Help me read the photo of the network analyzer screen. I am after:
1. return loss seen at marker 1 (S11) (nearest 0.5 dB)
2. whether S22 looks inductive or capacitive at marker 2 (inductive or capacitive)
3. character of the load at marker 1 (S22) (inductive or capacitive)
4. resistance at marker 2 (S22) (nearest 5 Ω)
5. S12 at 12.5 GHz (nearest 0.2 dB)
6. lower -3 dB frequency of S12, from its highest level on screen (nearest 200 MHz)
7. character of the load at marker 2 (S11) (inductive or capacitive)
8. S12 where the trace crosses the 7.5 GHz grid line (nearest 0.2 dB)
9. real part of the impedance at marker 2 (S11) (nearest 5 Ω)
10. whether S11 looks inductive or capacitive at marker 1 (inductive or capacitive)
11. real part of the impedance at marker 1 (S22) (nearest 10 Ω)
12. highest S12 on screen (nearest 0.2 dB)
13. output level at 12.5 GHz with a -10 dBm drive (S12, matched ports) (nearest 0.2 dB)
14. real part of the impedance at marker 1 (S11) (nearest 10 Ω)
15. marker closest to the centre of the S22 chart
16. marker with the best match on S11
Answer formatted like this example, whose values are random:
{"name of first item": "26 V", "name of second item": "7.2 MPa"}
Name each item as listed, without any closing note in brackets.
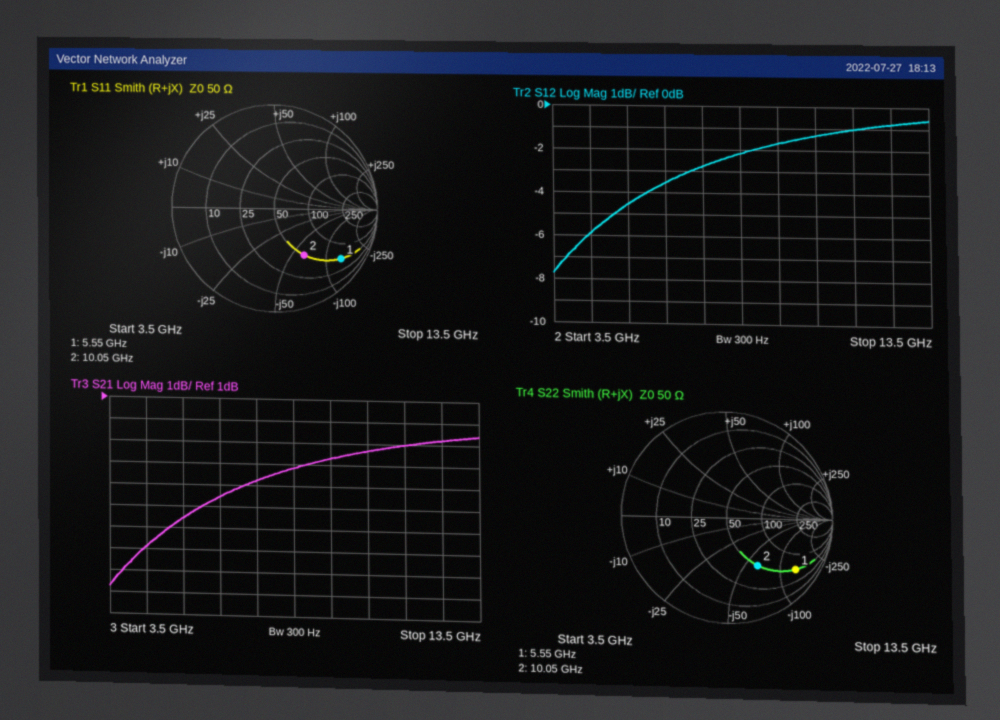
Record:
{"return loss seen at marker 1 (S11)": "2.0 dB", "whether S22 looks inductive or capacitive at marker 2": "capacitive", "character of the load at marker 1 (S22)": "capacitive", "resistance at marker 2 (S22)": "50 Ω", "S12 at 12.5 GHz": "-0.8 dB", "lower -3 dB frequency of S12, from its highest level on screen": "6.4 GHz", "character of the load at marker 2 (S11)": "capacitive", "S12 where the trace crosses the 7.5 GHz grid line": "-2.8 dB", "real part of the impedance at marker 2 (S11)": "50 Ω", "whether S11 looks inductive or capacitive at marker 1": "capacitive", "real part of the impedance at marker 1 (S22)": "50 Ω", "highest S12 on screen": "-0.6 dB", "output level at 12.5 GHz with a -10 dBm drive (S12, matched ports)": "-10.8 dBm", "real part of the impedance at marker 1 (S11)": "50 Ω", "marker closest to the centre of the S22 chart": "marker 2", "marker with the best match on S11": "marker 2"}
